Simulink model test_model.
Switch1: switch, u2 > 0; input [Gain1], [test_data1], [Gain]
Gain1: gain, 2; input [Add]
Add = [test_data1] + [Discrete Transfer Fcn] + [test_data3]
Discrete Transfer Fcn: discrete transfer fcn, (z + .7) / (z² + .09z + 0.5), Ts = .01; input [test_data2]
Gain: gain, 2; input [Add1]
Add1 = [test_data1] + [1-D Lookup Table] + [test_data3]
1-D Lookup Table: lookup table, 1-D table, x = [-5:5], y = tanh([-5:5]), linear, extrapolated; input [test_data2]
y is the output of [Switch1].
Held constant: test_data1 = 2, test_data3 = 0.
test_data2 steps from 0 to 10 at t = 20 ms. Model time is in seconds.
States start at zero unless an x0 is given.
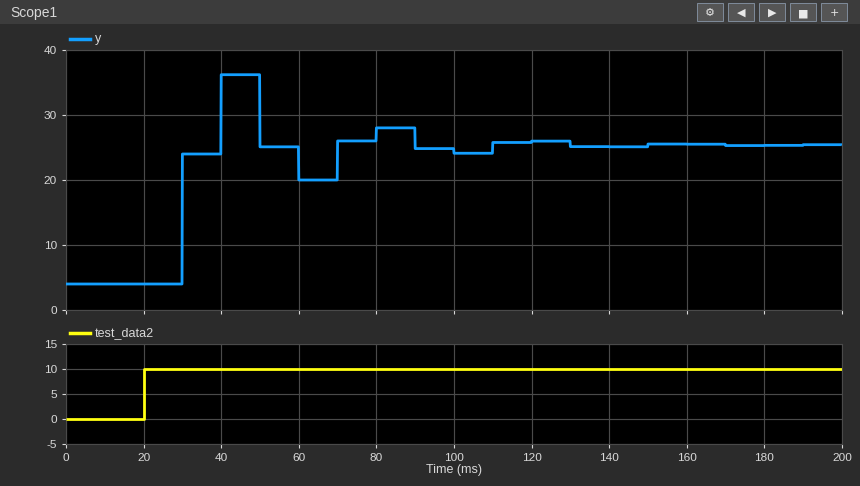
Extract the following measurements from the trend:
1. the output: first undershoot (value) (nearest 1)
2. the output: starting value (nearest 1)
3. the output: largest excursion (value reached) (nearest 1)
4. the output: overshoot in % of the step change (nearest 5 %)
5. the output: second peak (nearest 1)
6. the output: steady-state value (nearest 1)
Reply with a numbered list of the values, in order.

1. 20
2. 4
3. 36
4. 50 %
5. 28
6. 25
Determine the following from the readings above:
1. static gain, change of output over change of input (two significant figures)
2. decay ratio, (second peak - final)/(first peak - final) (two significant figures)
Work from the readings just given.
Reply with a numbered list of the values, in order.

1. 2.1
2. 0.27
